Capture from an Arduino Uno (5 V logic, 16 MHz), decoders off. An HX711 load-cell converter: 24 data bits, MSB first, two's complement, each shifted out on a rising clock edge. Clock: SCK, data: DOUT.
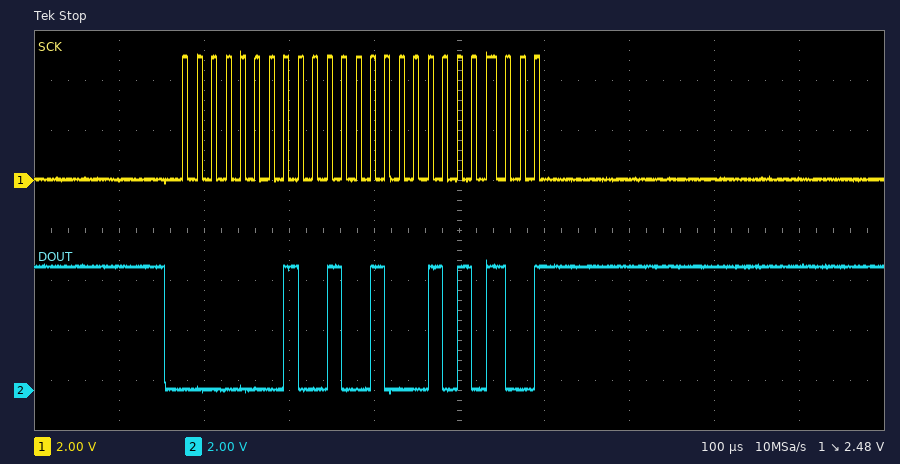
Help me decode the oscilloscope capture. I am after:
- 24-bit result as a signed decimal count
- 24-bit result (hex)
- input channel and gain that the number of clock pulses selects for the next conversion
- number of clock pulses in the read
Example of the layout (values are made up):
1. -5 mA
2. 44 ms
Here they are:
1. 74836
2. 0x012454
3. channel A, gain 128
4. 25
